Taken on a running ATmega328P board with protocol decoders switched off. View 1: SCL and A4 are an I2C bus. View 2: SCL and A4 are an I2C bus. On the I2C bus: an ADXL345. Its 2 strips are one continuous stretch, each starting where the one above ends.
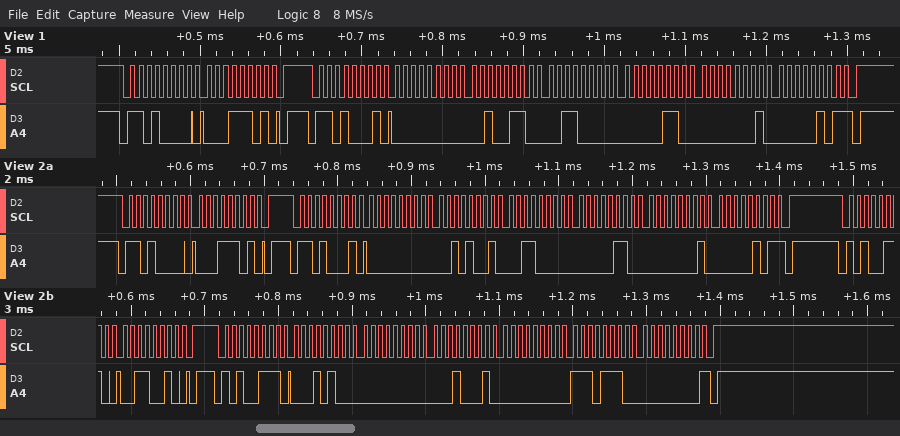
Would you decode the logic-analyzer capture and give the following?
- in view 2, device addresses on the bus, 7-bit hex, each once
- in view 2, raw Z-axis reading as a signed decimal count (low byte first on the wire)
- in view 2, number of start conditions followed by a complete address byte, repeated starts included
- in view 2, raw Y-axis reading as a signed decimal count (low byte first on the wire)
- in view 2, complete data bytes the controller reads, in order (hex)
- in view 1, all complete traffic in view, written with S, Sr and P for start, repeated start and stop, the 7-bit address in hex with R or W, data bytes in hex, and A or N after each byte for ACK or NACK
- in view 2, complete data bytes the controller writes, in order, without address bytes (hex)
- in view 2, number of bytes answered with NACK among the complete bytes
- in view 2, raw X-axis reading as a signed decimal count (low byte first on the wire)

0x68 0x53
238
4
17
00 29 30 06 01 05 14 00 11 00 EE 00
S 68W A 1D A P S 68R A 00 A 26 A 30 A 06 A 01 A 05 N P
1D 32
2
20
